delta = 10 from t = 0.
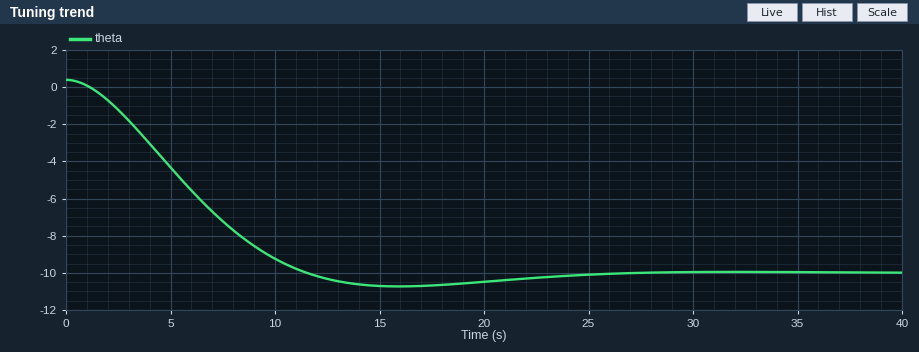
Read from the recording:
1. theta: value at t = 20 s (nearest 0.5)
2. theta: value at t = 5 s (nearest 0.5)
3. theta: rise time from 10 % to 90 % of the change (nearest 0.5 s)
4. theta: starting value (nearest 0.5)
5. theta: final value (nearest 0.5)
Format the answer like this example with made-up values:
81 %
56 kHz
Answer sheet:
-10.5
-4.5
7.5 s
0.5
-10.0
